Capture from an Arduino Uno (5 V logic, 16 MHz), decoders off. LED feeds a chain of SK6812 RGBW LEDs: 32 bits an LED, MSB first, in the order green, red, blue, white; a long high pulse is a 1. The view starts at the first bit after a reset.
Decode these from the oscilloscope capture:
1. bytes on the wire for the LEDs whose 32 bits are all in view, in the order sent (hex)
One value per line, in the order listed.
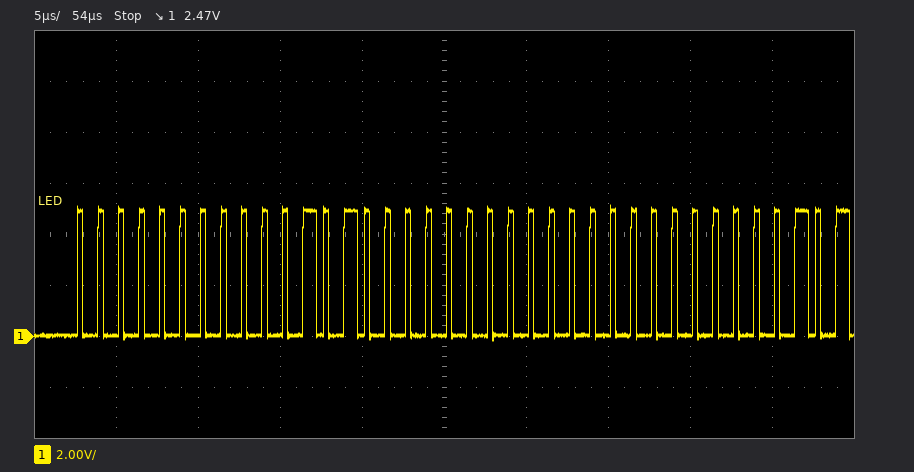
00 14 00 00
